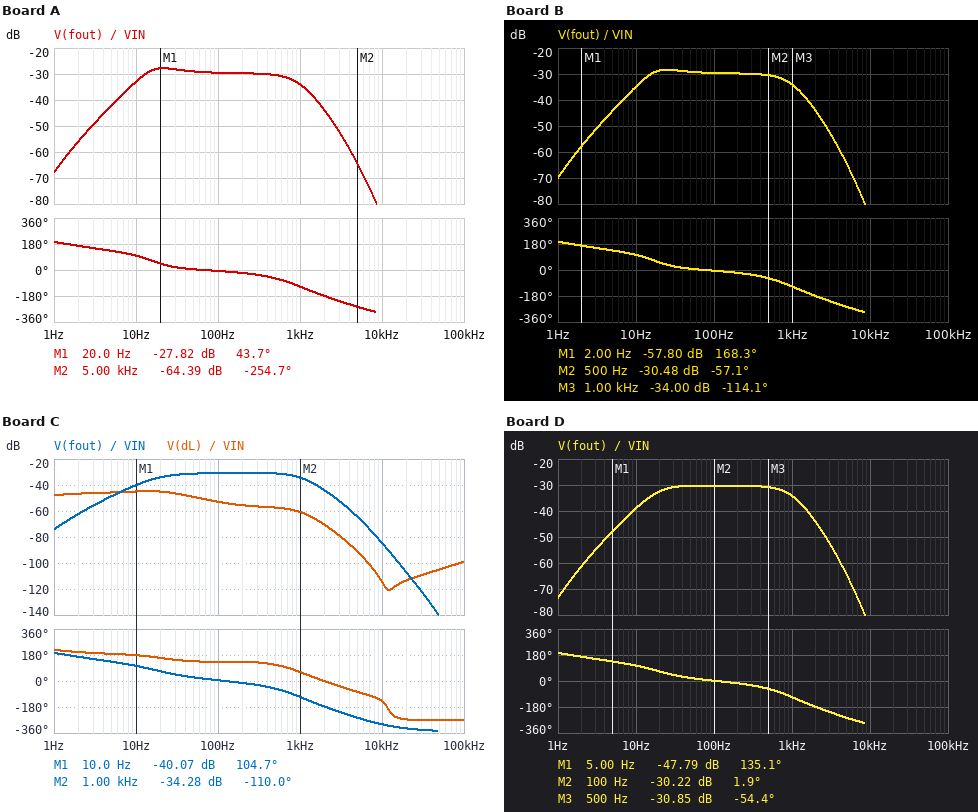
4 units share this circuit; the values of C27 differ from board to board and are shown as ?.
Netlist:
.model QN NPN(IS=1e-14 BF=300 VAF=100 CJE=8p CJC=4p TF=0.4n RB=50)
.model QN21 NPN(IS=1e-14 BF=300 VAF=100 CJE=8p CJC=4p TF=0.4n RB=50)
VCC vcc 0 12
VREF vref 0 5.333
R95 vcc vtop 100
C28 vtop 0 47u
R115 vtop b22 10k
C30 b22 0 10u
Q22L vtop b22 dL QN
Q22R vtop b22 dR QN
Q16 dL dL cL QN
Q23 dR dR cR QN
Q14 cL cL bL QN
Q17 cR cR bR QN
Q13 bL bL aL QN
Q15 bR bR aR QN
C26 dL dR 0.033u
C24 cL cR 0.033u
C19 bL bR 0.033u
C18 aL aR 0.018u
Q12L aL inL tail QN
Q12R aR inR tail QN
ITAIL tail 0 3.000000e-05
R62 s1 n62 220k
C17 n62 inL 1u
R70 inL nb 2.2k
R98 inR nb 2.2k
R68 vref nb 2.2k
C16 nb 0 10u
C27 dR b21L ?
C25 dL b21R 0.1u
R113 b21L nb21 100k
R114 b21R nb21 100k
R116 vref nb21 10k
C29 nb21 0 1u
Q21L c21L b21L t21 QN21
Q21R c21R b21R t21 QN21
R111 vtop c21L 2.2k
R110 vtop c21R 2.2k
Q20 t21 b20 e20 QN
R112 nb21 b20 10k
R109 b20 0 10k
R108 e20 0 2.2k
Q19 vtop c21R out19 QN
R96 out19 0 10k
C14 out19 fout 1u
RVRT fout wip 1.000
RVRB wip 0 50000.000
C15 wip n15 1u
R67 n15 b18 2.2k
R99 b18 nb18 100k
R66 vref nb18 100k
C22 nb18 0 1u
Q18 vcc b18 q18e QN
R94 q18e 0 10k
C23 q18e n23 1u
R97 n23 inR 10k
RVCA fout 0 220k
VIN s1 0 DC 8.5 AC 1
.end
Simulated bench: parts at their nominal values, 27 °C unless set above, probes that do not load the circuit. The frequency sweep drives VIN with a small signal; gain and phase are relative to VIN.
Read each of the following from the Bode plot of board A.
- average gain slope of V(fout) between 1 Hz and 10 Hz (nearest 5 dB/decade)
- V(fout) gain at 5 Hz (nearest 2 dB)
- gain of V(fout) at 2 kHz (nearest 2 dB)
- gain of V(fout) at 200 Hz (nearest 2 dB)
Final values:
35 dB/decade
-42 dB
-44 dB
-30 dB
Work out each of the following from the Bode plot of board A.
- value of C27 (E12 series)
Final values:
180 nF
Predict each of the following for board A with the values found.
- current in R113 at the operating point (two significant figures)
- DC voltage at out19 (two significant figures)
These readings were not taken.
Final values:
780 nA
11 V
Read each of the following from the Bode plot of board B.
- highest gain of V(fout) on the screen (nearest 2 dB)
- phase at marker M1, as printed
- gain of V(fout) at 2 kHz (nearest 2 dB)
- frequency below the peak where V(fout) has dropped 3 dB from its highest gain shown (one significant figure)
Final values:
-28 dB
168.3 deg
-44 dB
10 Hz
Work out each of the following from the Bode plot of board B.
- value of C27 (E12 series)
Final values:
120 nF
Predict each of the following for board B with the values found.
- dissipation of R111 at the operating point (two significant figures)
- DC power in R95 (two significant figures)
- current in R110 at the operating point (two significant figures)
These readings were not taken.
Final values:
140 µW
260 µW
260 µA
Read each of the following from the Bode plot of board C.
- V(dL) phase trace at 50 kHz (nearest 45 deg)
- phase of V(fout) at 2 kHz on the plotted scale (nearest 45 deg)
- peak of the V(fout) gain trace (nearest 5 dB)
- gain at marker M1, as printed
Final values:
-270 deg
-180 deg
-30 dB
-40.07 dB
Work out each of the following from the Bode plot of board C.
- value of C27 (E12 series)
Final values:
33 nF
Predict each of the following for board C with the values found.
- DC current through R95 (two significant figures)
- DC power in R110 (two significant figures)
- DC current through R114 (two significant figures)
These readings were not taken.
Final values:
1.6 mA
150 µW
780 nA
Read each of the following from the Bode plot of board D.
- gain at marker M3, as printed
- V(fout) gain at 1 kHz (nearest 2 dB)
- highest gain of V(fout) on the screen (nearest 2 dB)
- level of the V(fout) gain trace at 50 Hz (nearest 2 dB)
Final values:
-30.85 dB
-34 dB
-30 dB
-30 dB
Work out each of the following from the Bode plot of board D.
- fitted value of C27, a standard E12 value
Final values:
47 nF
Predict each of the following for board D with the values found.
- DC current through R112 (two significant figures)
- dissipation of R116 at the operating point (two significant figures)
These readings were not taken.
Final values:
180 µA
320 µW
